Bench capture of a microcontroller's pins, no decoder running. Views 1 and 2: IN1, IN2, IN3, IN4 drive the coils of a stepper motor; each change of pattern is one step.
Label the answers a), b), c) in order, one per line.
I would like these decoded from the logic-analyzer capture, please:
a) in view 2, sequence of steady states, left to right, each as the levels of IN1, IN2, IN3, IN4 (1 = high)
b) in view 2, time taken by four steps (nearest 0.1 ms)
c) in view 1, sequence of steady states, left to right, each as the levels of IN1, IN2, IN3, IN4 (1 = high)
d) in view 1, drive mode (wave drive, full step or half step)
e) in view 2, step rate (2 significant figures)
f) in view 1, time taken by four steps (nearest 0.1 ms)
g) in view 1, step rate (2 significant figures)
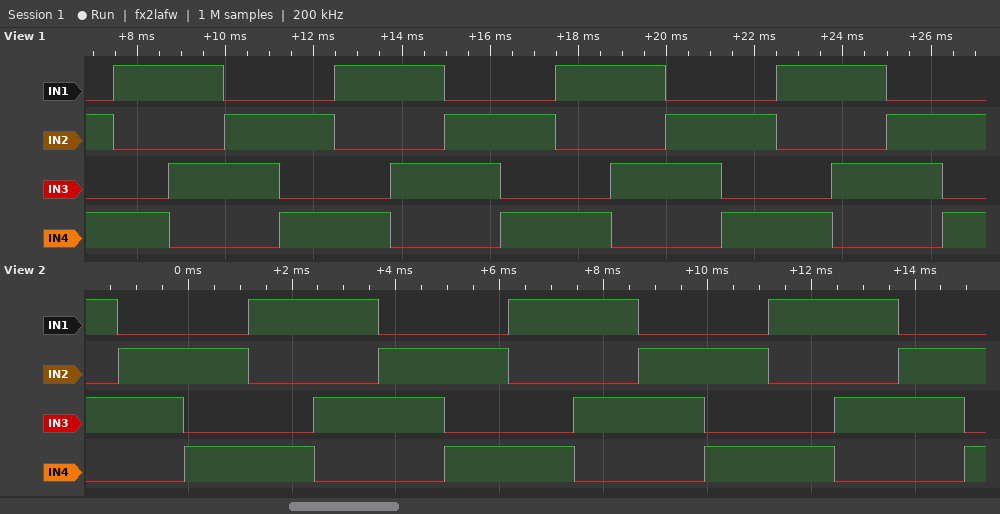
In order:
a) 1010 0110 0101 1001 1010 0110 0101 1001 1010 0110 0101 1001 1010 0110 0101
b) 5.0 ms
c) 0101 1001 1010 0110 0101 1001 1010 0110 0101 1001 1010 0110 0101 1001 1010 0110 0101
d) full step
e) 800 steps/s
f) 5.0 ms
g) 800 steps/s
